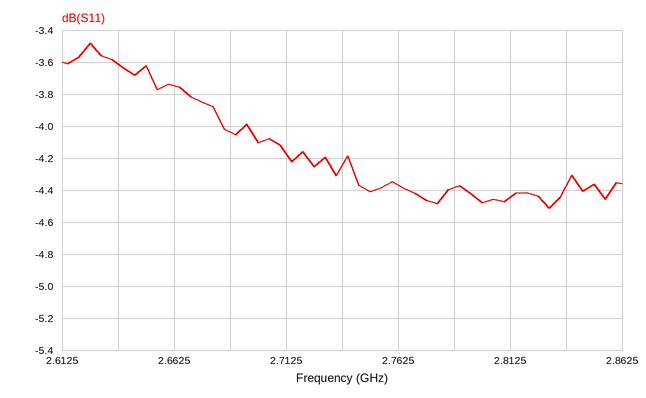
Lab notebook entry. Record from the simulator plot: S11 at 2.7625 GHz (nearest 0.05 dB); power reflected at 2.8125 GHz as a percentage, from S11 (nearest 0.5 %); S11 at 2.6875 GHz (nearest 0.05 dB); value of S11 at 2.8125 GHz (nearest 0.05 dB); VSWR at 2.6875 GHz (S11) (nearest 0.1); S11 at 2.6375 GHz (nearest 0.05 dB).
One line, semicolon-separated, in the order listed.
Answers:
-4.35 dB; 36.0 %; -4.05 dB; -4.45 dB; 4.4; -3.60 dB
